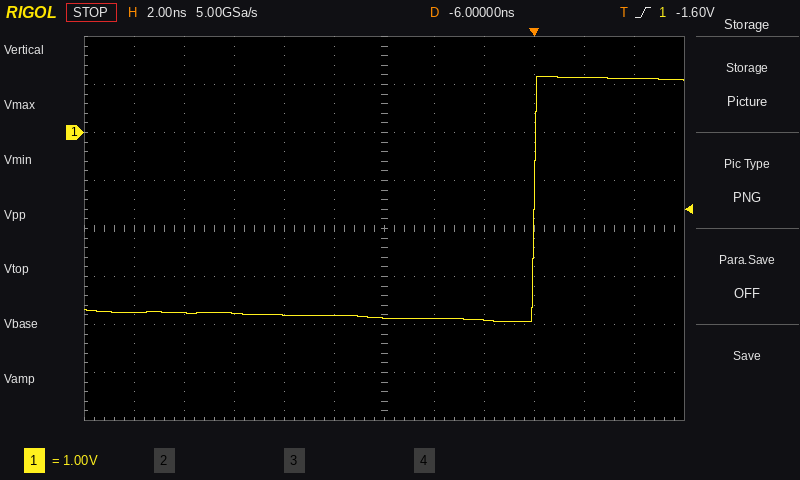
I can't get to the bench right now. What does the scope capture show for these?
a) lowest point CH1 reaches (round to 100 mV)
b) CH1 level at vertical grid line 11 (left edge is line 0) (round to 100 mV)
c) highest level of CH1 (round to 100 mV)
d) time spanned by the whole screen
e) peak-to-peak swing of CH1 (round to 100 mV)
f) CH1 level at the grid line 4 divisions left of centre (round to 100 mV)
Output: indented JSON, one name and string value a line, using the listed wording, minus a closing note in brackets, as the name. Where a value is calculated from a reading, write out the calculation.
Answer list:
{
  "lowest point CH1 reaches": "-3.9 V",
  "CH1 level at vertical grid line 11 (left edge is line 0)": "1.1 V",
  "highest level of CH1": "1.2 V",
  "time spanned by the whole screen": "24 ns",
  "peak-to-peak swing of CH1": "1.2 V − (-3.9 V) = 5.1 V",
  "CH1 level at the grid line 4 divisions left of centre": "-3.8 V"
}
